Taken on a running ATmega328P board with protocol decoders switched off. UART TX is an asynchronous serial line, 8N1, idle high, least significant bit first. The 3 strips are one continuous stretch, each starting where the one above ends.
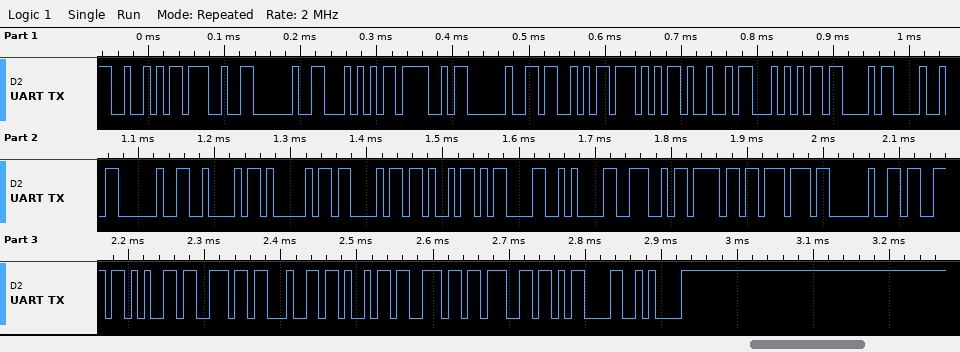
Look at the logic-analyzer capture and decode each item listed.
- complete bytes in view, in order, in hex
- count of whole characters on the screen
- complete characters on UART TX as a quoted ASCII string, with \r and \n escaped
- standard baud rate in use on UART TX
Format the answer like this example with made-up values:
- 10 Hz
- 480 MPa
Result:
- 52 27 20 54 4F 20 53 57 49 54 43 48 20 42 41 43 4B 0D 0A 4E 6F 77 20 73 65 6E 64 69 6E 67 0D 0A
- 32
- "R' TO SWITCH BACK\r\nNow sending\r\n"
- 115200 baud
